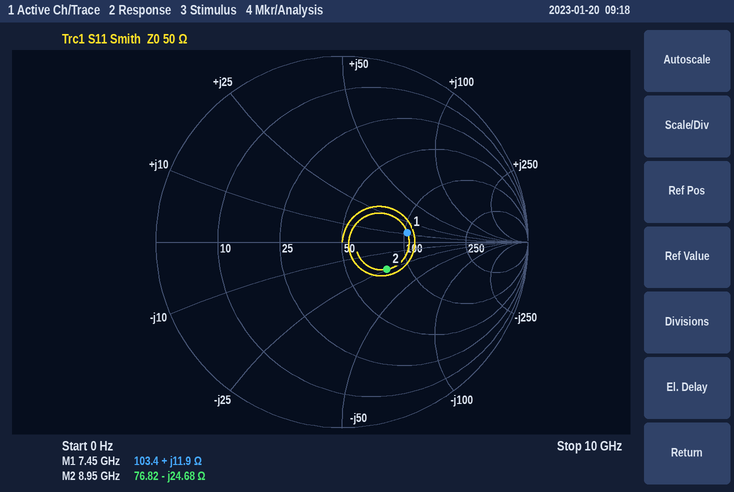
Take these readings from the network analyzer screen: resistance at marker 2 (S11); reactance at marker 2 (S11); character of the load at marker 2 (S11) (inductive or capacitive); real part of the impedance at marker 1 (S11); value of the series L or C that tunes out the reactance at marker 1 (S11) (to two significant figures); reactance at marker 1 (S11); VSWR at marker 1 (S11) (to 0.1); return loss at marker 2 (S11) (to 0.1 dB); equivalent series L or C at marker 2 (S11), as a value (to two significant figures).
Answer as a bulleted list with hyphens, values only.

- 76.82 Ω
- -24.68 Ω
- capacitive
- 103.4 Ω
- 1.8 pF
- +11.9 Ω
- 2.1
- 11.0 dB
- 720 fF
